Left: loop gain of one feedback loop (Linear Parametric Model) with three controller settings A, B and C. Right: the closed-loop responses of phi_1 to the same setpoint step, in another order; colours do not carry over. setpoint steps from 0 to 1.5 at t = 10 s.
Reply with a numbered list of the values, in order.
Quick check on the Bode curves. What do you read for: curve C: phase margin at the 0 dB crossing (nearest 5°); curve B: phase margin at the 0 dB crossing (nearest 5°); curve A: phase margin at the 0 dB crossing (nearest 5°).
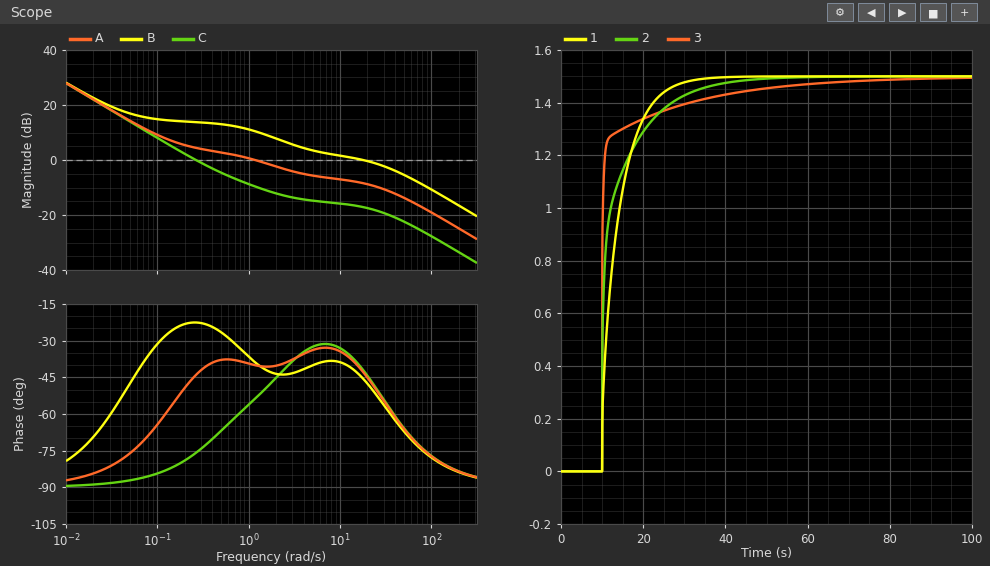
1. 105°
2. 135°
3. 140°
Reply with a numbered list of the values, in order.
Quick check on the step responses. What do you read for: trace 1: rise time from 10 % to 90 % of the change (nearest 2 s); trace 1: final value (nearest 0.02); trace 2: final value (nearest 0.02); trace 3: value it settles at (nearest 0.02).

1. 10 s
2. 1.50
3. 1.50
4. 1.50
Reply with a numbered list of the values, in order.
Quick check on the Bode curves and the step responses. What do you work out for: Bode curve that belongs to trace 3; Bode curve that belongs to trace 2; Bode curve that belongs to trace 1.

1. B
2. A
3. C
